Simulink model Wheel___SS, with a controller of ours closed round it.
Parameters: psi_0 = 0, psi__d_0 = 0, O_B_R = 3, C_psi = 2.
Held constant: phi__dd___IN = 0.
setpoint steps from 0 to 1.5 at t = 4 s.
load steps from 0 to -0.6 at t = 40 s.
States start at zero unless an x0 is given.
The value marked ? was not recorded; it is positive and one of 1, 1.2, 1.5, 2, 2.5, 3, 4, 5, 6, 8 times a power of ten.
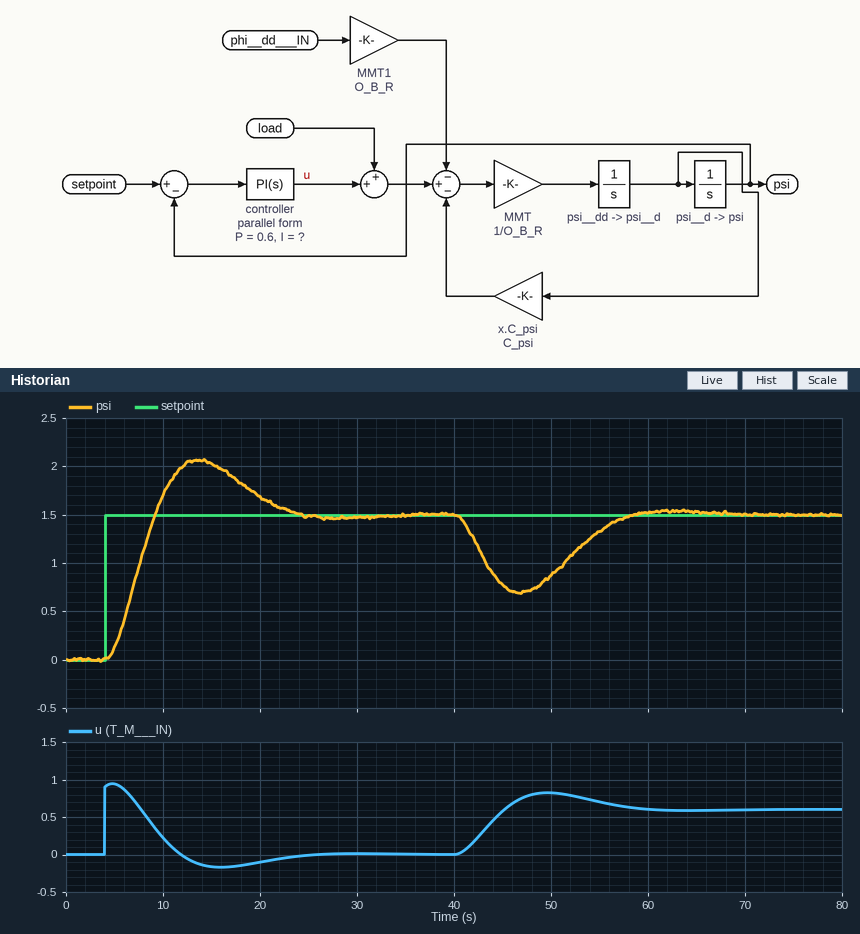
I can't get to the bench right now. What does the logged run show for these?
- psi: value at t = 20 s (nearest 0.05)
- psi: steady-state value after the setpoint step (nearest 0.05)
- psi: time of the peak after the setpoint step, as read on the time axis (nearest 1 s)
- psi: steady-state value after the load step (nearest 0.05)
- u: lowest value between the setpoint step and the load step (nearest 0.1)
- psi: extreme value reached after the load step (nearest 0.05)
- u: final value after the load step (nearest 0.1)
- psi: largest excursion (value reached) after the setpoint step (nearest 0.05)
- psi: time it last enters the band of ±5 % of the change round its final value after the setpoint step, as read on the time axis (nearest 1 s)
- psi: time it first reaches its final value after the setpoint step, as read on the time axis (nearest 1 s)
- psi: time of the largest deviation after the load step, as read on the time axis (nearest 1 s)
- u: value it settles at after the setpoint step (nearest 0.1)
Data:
1.70
1.50
14 s
1.50
-0.2
0.70
0.6
2.05
22 s
9 s
47 s
0.0
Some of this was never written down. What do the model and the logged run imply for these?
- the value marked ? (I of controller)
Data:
0.08
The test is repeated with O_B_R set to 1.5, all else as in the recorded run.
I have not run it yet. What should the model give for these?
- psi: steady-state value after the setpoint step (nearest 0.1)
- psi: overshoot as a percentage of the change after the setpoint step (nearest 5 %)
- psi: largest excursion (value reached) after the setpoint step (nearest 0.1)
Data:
1.5
25 %
1.9
